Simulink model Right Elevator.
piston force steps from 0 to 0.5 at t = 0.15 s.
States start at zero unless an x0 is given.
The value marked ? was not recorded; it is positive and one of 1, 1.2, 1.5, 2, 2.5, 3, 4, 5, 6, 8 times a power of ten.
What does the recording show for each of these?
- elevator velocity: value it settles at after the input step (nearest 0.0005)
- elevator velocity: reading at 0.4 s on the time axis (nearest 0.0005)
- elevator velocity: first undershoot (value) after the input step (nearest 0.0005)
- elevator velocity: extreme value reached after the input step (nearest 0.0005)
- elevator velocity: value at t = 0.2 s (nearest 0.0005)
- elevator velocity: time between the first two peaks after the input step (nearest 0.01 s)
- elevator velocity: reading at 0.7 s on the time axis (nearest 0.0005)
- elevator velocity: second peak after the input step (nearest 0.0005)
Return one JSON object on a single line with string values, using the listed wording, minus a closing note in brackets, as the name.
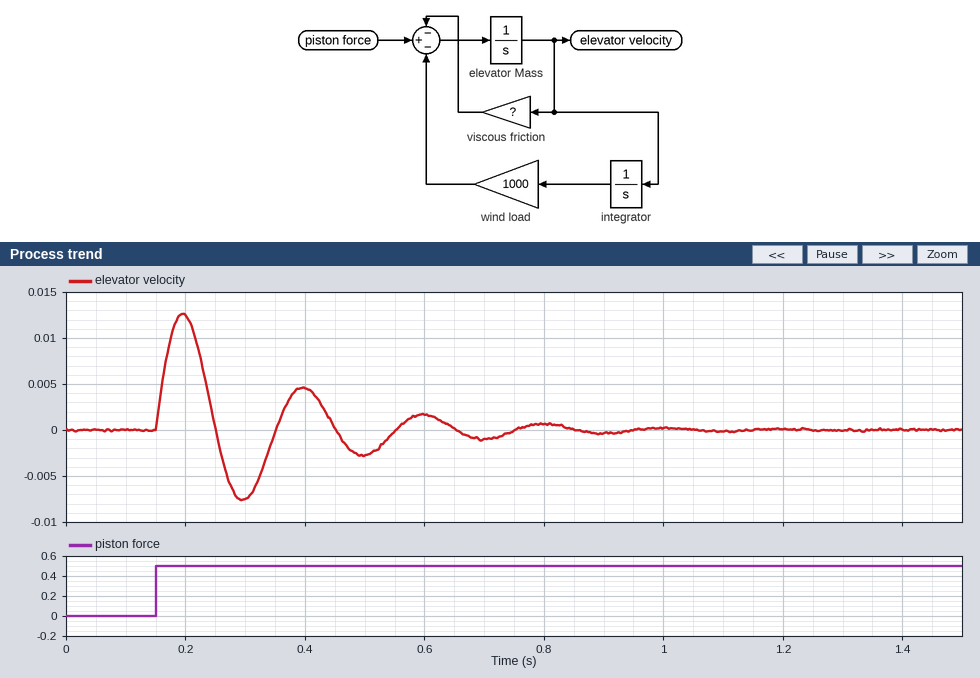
{"elevator velocity: value it settles at after the input step": "0.0000", "elevator velocity: reading at 0.4 s on the time axis": "0.0045", "elevator velocity: first undershoot (value) after the input step": "-0.0075", "elevator velocity: extreme value reached after the input step": "0.0125", "elevator velocity: value at t = 0.2 s": "0.0125", "elevator velocity: time between the first two peaks after the input step": "0.20 s", "elevator velocity: reading at 0.7 s on the time axis": "-0.0010", "elevator velocity: second peak after the input step": "0.0045"}
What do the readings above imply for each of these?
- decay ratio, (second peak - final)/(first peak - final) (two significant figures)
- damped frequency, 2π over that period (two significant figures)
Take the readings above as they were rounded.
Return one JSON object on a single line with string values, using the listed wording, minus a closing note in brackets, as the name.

{"decay ratio, (second peak - final)/(first peak - final)": "0.36", "damped frequency, 2π over that period": "31 rad/s"}
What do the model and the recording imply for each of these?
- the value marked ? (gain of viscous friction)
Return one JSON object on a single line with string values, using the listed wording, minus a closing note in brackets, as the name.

{"the value marked ?": "10"}
